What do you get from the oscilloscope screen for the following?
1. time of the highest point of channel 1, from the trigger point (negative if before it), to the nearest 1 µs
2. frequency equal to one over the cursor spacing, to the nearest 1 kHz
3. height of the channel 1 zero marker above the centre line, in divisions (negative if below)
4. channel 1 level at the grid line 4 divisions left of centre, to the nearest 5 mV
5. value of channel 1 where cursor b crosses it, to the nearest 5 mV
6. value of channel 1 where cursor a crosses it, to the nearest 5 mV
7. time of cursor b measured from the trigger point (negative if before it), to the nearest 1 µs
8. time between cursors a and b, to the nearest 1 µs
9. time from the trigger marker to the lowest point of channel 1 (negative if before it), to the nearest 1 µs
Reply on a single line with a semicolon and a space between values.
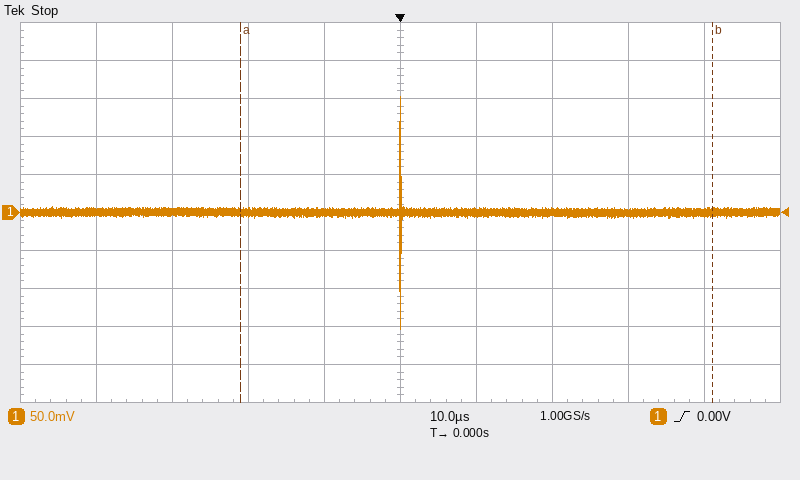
0 µs; 16 kHz; 0.0 div; 0 mV; 0 mV; 0 mV; +41 µs; 62 µs; 0 µs
